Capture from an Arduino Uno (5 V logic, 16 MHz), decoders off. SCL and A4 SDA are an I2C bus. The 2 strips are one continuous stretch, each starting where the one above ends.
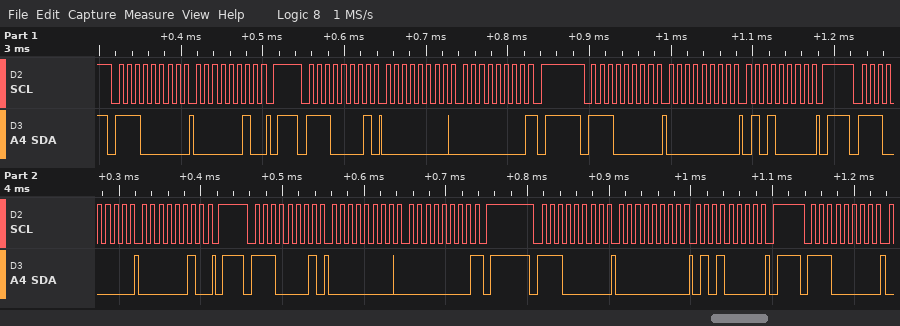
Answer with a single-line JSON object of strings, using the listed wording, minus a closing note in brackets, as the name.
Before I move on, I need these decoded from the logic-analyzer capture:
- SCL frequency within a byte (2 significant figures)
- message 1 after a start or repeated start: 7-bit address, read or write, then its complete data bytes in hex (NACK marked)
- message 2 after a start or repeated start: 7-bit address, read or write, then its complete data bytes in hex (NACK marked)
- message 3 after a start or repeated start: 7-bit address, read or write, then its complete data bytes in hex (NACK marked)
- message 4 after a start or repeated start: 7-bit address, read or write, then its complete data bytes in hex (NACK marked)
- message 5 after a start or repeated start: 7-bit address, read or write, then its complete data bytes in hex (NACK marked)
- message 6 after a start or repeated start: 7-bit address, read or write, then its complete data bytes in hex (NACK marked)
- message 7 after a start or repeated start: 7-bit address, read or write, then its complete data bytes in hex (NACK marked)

{"SCL frequency within a byte": "100 kHz", "message 1 after a start or repeated start: 7-bit address, read or write, then its complete data bytes in hex": "0x70 write: 02", "message 2 after a start or repeated start: 7-bit address, read or write, then its complete data bytes in hex": "0x70 read: 00 00 NACK", "message 3 after a start or repeated start: 7-bit address, read or write, then its complete data bytes in hex": "0x70 write: 00 50", "message 4 after a start or repeated start: 7-bit address, read or write, then its complete data bytes in hex": "0x70 write: 02", "message 5 after a start or repeated start: 7-bit address, read or write, then its complete data bytes in hex": "0x70 read: 00 00 NACK", "message 6 after a start or repeated start: 7-bit address, read or write, then its complete data bytes in hex": "0x70 write: 00 50", "message 7 after a start or repeated start: 7-bit address, read or write, then its complete data bytes in hex": "0x70 write"}
